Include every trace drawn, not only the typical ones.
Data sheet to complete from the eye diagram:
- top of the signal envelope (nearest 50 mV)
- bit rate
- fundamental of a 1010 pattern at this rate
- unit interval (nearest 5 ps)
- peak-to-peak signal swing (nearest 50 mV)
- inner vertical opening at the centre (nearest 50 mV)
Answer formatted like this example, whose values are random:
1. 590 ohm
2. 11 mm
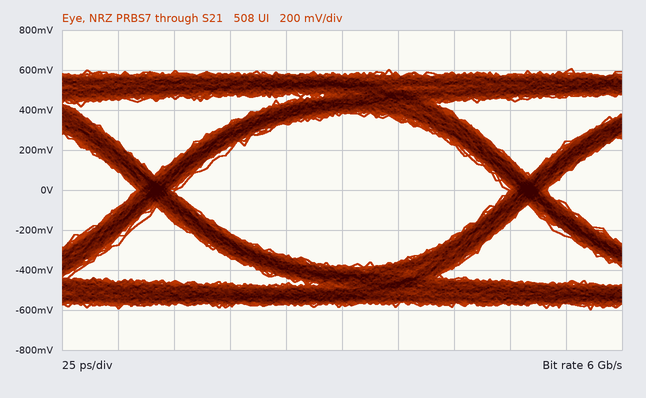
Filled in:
1. 600 mV
2. 6 Gb/s
3. 3 GHz
4. 165 ps
5. 1.20 V
6. 750 mV
